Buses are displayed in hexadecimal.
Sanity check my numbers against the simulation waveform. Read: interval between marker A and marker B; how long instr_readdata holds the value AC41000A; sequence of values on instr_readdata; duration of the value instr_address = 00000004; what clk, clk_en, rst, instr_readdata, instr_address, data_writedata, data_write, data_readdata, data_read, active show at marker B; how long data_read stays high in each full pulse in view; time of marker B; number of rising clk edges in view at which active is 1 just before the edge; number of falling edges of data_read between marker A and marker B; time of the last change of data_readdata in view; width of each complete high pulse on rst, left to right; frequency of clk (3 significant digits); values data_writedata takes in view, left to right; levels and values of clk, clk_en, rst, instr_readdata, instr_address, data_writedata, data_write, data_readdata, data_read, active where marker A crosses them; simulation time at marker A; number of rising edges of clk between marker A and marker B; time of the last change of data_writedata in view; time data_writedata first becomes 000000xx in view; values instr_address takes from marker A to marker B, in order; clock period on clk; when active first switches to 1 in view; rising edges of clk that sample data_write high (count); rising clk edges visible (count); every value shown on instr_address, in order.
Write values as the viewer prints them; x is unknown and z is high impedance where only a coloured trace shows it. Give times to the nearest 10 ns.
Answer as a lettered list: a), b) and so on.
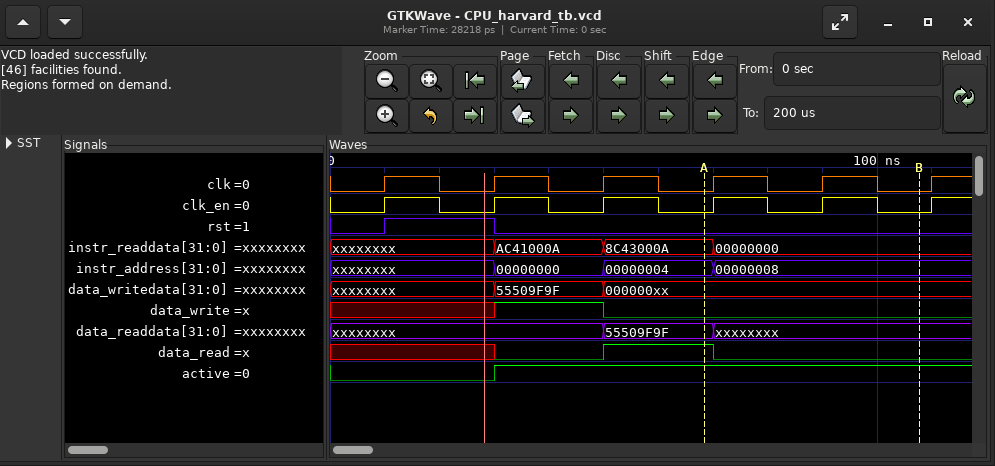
a) 40 ns
b) 20 ns
c) xxxxxxxx, AC41000A, 8C43000A, 00000000
d) 20 ns
e) clk=0, clk_en=0, rst=0, instr_readdata=00000000, instr_address=00000008, data_writedata=000000xx, data_write=0, data_readdata=xxxxxxxx, data_read=0, active=1
f) 20 ns
g) 110 ns
h) 4
i) 1
j) 70 ns
k) 20 ns
l) 50.0 MHz
m) xxxxxxxx, 55509F9F, 000000xx
n) clk=0, clk_en=0, rst=0, instr_readdata=8C43000A, instr_address=00000004, data_writedata=000000xx, data_write=0, data_readdata=55509F9F, data_read=1, active=1
o) 70 ns
p) 2
q) 50 ns
r) 50 ns
s) 00000004, 00000008
t) 20 ns
u) 30 ns
v) 1
w) 6
x) xxxxxxxx, 00000000, 00000004, 00000008
